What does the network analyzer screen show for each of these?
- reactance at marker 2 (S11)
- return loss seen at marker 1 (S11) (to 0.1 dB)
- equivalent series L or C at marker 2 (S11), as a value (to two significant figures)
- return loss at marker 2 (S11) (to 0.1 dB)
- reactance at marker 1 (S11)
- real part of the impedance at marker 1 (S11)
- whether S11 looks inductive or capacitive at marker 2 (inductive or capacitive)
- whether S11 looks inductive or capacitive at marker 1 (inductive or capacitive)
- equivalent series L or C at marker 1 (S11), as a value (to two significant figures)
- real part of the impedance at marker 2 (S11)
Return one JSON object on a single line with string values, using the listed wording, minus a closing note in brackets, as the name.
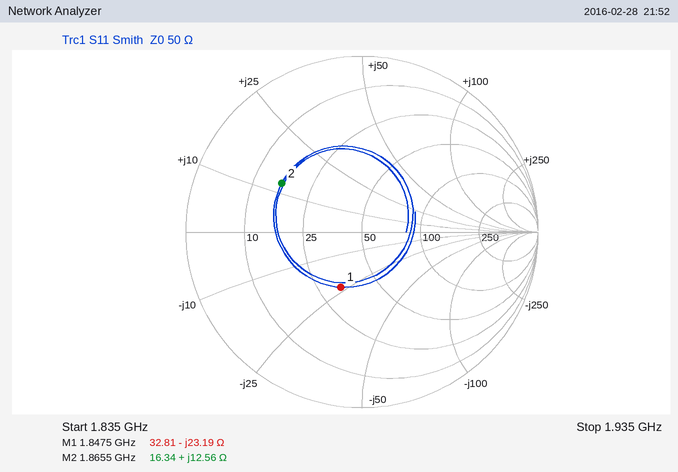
{"reactance at marker 2": "+12.56 Ω", "return loss seen at marker 1 (S11)": "9.5 dB", "equivalent series L or C at marker 2 (S11), as a value": "1.1 nH", "return loss at marker 2 (S11)": "5.5 dB", "reactance at marker 1": "-23.19 Ω", "real part of the impedance at marker 1": "32.81 Ω", "whether S11 looks inductive or capacitive at marker 2": "inductive", "whether S11 looks inductive or capacitive at marker 1": "capacitive", "equivalent series L or C at marker 1 (S11), as a value": "3.7 pF", "real part of the impedance at marker 2": "16.34 Ω"}
